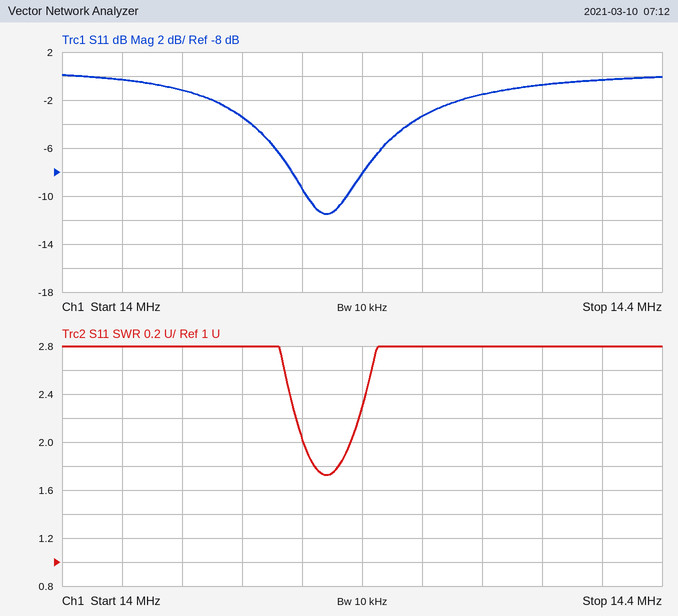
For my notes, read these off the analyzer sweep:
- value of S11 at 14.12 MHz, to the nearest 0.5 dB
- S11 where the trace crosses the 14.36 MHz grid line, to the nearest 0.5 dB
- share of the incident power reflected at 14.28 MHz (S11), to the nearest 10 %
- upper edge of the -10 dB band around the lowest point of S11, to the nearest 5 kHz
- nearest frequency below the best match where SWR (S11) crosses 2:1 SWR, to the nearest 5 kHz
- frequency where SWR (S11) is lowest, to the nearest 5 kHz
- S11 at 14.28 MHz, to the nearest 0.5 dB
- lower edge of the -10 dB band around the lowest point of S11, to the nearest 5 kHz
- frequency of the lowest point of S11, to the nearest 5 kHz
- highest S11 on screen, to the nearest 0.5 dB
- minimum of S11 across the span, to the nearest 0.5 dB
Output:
-3.5 dB
-0.5 dB
70 %
14.190 MHz
14.160 MHz
14.175 MHz
-1.5 dB
14.165 MHz
14.175 MHz
0.0 dB
-11.5 dB
